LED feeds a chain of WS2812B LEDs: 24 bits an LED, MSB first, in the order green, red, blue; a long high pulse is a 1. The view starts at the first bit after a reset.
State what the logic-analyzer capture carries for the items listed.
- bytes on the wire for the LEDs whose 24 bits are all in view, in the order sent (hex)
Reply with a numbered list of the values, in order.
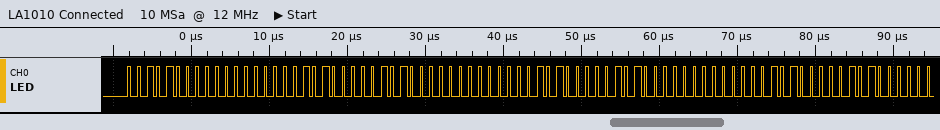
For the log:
1. 28 00 28 28 00 28 28 00 28
